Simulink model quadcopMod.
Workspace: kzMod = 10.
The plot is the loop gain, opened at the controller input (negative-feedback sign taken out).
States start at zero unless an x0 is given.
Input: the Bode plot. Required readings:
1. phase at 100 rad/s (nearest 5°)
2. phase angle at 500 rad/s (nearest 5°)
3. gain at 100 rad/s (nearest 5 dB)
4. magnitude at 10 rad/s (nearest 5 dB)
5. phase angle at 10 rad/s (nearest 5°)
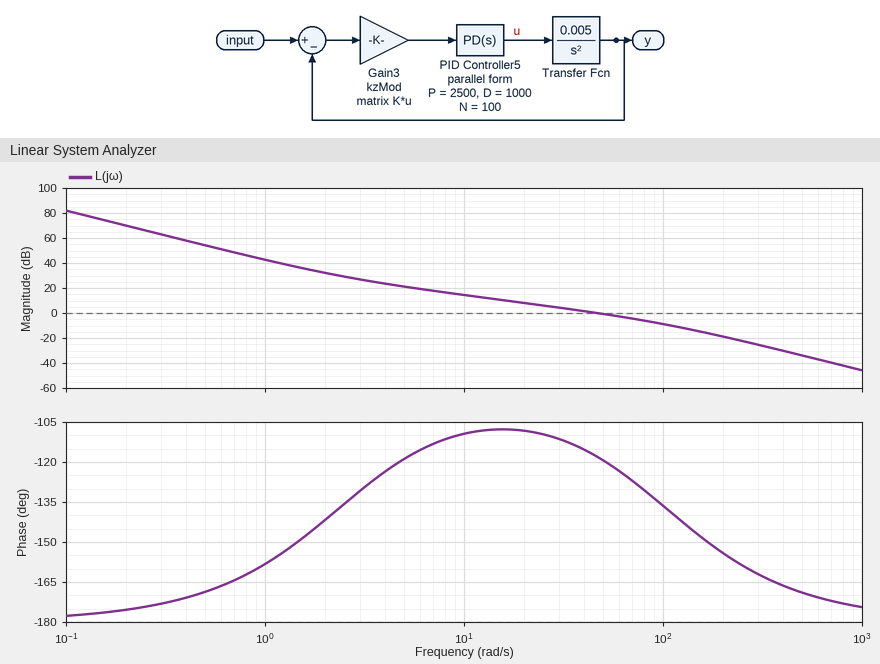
-135°
-170°
-10 dB
15 dB
-110°
